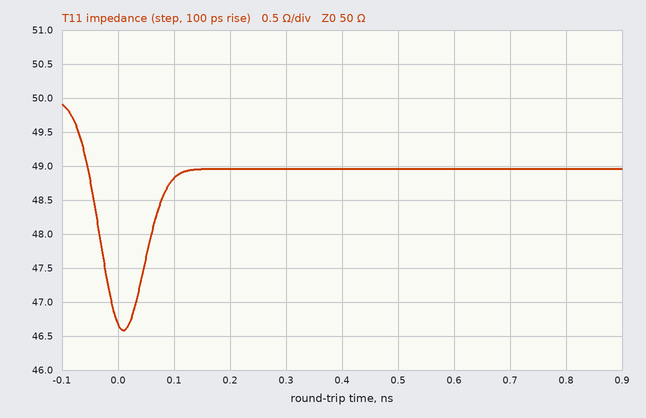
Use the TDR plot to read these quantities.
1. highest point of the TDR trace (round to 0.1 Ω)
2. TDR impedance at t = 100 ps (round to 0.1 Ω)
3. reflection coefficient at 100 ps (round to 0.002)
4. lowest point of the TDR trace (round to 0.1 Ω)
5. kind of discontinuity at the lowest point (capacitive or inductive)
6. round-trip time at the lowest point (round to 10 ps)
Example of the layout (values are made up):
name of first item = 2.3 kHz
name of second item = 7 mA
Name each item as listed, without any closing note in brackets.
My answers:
highest point of the TDR trace = 49.9 Ω
TDR impedance at t = 100 ps = 48.8 Ω
reflection coefficient at 100 ps = -0.012
lowest point of the TDR trace = 46.6 Ω
kind of discontinuity at the lowest point = capacitive
round-trip time at the lowest point = 10 ps
